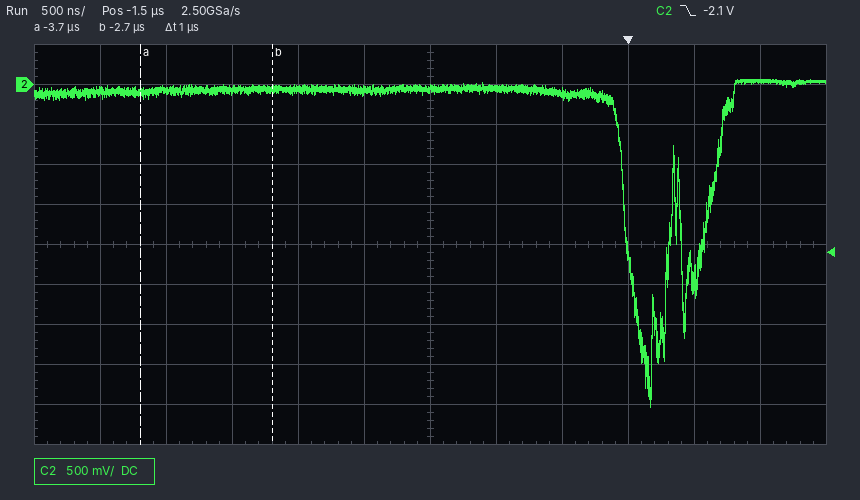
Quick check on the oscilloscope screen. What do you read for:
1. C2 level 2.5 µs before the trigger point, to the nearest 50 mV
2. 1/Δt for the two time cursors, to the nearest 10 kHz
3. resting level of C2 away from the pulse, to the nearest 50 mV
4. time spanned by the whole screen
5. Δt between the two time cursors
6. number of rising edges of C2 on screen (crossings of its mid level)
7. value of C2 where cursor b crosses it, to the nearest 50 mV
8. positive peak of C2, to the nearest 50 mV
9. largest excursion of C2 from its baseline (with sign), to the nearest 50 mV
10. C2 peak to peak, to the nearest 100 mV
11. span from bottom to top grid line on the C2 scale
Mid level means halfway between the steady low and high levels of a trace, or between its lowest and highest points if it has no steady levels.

-50 mV
1.00 MHz
-50 mV
6 µs
1 µs
2
-50 mV
50 mV
-3.95 V
4.10 V
5 V
